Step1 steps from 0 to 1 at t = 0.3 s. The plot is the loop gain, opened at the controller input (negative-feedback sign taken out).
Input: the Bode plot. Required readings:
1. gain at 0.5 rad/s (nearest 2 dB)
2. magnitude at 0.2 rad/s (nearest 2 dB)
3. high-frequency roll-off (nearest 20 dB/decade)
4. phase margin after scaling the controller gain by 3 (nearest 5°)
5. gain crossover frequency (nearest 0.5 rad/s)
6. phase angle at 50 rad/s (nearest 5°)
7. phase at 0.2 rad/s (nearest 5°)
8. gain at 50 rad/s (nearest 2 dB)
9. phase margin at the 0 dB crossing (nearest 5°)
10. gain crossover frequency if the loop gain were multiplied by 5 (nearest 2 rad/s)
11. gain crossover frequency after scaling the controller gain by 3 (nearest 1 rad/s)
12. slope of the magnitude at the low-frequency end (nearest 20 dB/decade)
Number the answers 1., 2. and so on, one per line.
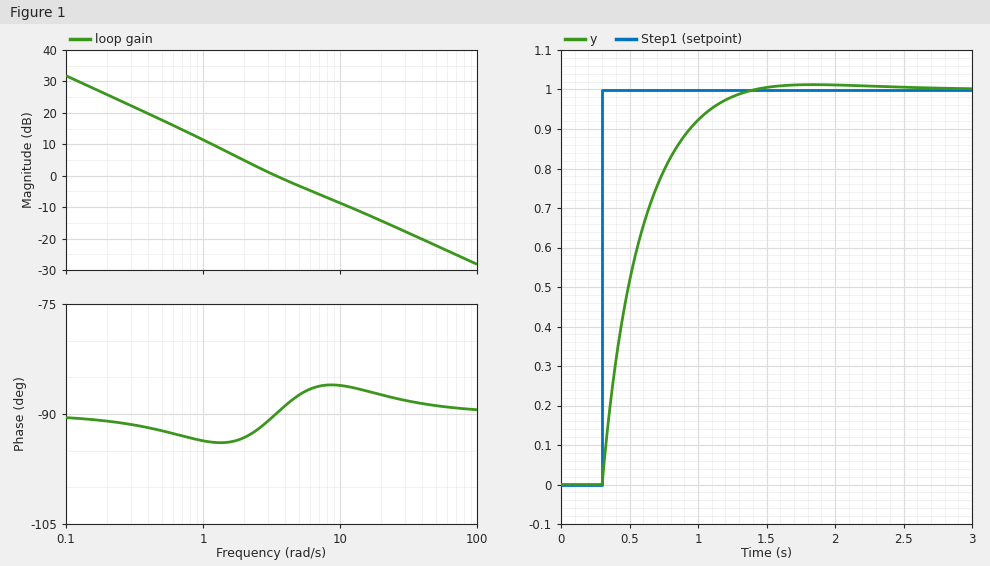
1. 18 dB
2. 26 dB
3. -20 dB/decade
4. 95°
5. 3.5 rad/s
6. -90°
7. -90°
8. -22 dB
9. 90°
10. 20 rad/s
11. 11 rad/s
12. -20 dB/decade
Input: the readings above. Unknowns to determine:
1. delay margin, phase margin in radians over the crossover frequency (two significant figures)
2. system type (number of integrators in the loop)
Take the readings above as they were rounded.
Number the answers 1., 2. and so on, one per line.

1. 0.45 s
2. 1
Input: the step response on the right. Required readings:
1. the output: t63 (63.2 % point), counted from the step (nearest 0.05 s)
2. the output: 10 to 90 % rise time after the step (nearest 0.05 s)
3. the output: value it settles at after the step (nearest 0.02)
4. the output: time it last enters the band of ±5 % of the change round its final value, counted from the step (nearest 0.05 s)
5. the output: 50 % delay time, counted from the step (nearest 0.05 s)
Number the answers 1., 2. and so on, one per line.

1. 0.30 s
2. 0.60 s
3. 1.00
4. 0.80 s
5. 0.20 s
